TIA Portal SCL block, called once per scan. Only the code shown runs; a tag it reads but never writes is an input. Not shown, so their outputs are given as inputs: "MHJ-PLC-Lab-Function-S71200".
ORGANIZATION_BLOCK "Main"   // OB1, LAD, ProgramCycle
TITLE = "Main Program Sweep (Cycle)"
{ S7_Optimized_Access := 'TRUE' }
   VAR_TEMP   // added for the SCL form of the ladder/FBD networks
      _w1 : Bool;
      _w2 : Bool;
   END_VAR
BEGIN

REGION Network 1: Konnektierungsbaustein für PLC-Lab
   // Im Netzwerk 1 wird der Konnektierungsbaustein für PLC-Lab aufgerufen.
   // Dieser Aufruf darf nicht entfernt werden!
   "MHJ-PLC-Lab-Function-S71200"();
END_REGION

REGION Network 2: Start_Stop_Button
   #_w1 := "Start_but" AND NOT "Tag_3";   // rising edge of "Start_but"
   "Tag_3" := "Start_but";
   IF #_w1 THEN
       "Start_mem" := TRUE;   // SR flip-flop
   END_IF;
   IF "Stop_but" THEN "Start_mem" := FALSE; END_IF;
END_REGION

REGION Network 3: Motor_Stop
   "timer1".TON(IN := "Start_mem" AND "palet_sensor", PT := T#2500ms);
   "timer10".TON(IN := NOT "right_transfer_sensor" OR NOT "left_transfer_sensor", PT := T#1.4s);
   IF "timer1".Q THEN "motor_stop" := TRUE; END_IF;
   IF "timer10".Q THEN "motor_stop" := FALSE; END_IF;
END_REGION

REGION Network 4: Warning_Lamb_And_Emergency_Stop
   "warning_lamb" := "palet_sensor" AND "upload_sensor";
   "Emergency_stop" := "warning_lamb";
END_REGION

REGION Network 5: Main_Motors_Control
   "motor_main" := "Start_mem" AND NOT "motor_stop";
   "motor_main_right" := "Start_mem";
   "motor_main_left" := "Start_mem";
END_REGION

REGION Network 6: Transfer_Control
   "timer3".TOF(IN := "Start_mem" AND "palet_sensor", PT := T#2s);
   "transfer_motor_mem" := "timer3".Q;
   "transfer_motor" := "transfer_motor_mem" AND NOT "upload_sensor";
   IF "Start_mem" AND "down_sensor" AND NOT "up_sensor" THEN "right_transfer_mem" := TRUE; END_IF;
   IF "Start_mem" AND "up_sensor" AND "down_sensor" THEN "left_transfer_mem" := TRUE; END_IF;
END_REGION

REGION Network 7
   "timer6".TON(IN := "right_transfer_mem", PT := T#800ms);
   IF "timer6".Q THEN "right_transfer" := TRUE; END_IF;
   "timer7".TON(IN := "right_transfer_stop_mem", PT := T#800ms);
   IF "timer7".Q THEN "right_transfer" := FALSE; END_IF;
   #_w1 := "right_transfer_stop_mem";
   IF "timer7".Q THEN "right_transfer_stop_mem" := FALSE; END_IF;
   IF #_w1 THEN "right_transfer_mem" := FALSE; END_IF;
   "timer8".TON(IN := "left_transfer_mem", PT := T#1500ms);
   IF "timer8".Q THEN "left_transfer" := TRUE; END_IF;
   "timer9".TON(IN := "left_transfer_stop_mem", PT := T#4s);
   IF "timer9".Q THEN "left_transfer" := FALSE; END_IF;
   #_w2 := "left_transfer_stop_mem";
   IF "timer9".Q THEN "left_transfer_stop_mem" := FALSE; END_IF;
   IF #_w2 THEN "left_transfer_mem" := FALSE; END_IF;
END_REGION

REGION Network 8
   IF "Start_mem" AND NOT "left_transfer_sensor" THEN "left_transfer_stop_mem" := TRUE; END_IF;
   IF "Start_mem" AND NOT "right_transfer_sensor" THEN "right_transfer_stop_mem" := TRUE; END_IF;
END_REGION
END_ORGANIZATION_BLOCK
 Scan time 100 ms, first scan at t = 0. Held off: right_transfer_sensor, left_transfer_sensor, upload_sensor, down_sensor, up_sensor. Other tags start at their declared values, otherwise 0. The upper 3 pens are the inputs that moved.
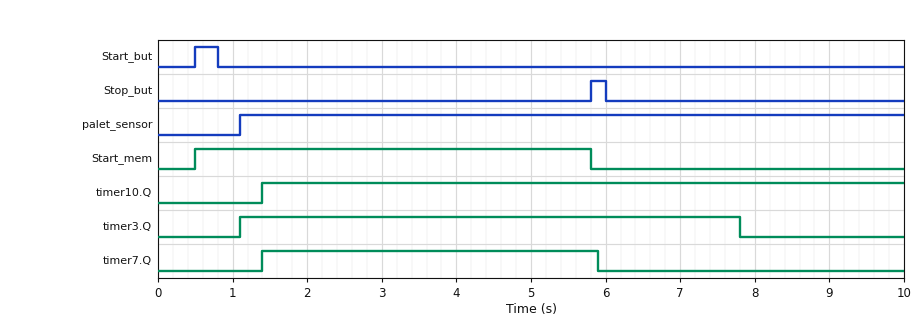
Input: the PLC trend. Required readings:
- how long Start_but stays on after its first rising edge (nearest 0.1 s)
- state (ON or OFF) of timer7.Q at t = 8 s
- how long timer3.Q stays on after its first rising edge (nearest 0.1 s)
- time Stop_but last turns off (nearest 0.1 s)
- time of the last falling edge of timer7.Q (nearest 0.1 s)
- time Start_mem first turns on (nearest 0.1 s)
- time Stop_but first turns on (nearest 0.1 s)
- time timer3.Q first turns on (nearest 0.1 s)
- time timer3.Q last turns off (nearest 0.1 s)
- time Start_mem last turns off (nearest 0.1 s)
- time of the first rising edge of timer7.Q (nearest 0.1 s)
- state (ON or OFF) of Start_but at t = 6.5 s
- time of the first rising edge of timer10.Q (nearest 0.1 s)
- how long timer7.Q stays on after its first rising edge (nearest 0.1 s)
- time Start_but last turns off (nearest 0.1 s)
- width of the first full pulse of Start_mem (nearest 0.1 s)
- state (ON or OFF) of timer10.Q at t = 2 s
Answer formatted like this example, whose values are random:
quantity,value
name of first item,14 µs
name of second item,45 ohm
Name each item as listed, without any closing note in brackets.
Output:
quantity,value
how long Start_but stays on after its first rising edge,0.3 s
state (ON or OFF) of timer7.Q at t = 8 s,OFF
how long timer3.Q stays on after its first rising edge,6.7 s
time Stop_but last turns off,6.0 s
time of the last falling edge of timer7.Q,5.9 s
time Start_mem first turns on,0.5 s
time Stop_but first turns on,5.8 s
time timer3.Q first turns on,1.1 s
time timer3.Q last turns off,7.8 s
time Start_mem last turns off,5.8 s
time of the first rising edge of timer7.Q,1.4 s
state (ON or OFF) of Start_but at t = 6.5 s,OFF
time of the first rising edge of timer10.Q,1.4 s
how long timer7.Q stays on after its first rising edge,4.5 s
time Start_but last turns off,0.8 s
width of the first full pulse of Start_mem,5.3 s
state (ON or OFF) of timer10.Q at t = 2 s,ON
